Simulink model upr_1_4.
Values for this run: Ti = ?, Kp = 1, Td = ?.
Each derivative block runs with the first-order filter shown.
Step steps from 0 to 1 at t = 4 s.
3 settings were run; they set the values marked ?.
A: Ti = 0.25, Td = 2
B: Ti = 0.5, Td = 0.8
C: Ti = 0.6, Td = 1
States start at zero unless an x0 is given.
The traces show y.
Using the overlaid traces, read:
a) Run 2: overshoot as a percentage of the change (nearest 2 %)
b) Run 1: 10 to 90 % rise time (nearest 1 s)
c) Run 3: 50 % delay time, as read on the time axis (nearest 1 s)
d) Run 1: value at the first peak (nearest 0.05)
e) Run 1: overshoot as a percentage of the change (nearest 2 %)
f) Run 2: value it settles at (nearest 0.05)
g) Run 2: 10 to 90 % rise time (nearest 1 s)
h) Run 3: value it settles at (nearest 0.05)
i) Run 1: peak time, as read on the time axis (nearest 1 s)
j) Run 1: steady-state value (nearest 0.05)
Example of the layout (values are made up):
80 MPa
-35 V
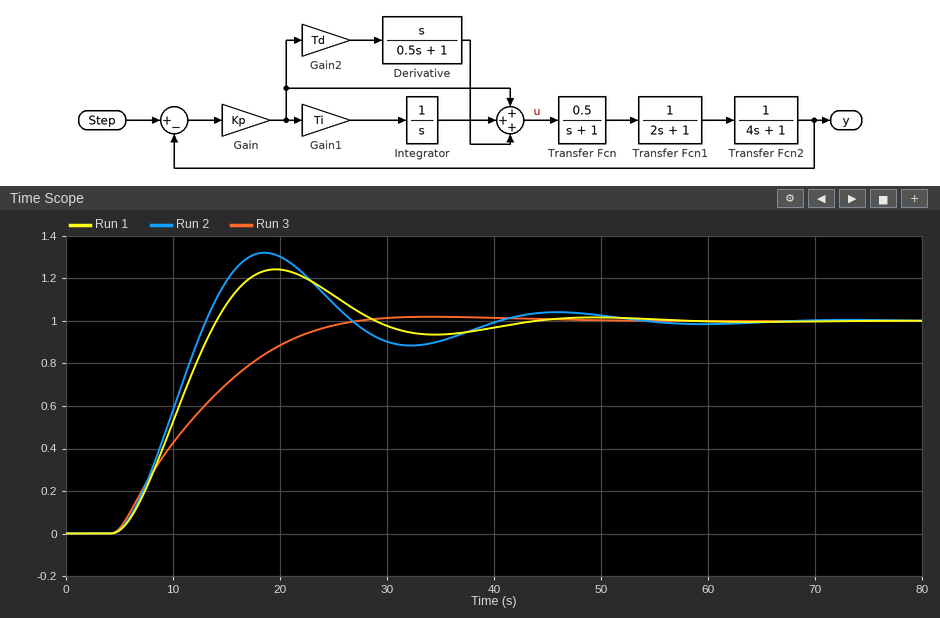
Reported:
32 %
7 s
11 s
1.25
24 %
1.00
6 s
1.00
20 s
1.00
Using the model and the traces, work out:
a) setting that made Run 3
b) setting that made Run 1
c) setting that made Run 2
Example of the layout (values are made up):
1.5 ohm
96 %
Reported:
A
B
C
